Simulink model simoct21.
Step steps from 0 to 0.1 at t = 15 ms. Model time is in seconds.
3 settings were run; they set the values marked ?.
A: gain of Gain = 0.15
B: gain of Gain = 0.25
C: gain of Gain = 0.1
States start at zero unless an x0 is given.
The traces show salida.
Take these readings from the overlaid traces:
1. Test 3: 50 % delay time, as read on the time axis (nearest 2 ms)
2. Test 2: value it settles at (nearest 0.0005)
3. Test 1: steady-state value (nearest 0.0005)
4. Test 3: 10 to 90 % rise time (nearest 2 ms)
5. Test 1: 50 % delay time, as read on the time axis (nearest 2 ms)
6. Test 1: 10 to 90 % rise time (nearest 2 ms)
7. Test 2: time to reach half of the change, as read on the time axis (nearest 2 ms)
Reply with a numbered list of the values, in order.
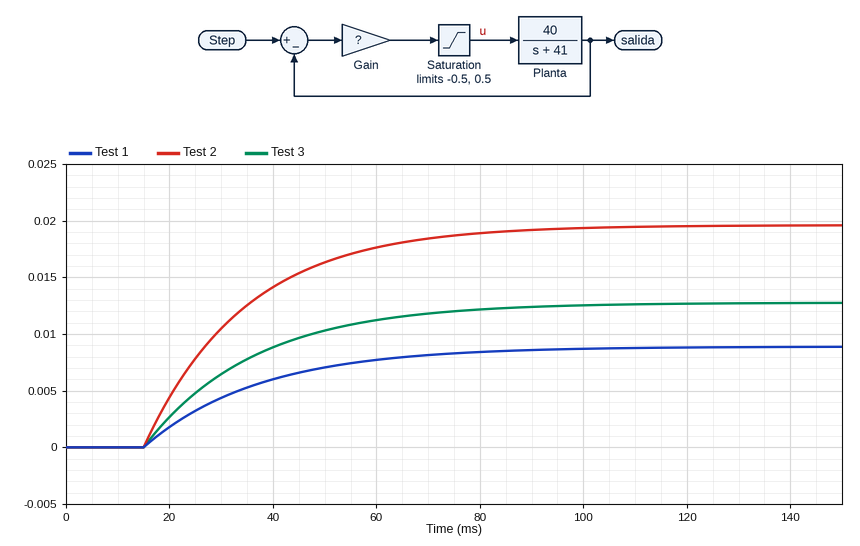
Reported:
1. 30 ms
2. 0.0195
3. 0.0090
4. 46 ms
5. 30 ms
6. 48 ms
7. 28 ms
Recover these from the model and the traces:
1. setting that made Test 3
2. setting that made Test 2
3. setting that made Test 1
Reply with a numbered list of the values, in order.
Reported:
1. A
2. B
3. C
